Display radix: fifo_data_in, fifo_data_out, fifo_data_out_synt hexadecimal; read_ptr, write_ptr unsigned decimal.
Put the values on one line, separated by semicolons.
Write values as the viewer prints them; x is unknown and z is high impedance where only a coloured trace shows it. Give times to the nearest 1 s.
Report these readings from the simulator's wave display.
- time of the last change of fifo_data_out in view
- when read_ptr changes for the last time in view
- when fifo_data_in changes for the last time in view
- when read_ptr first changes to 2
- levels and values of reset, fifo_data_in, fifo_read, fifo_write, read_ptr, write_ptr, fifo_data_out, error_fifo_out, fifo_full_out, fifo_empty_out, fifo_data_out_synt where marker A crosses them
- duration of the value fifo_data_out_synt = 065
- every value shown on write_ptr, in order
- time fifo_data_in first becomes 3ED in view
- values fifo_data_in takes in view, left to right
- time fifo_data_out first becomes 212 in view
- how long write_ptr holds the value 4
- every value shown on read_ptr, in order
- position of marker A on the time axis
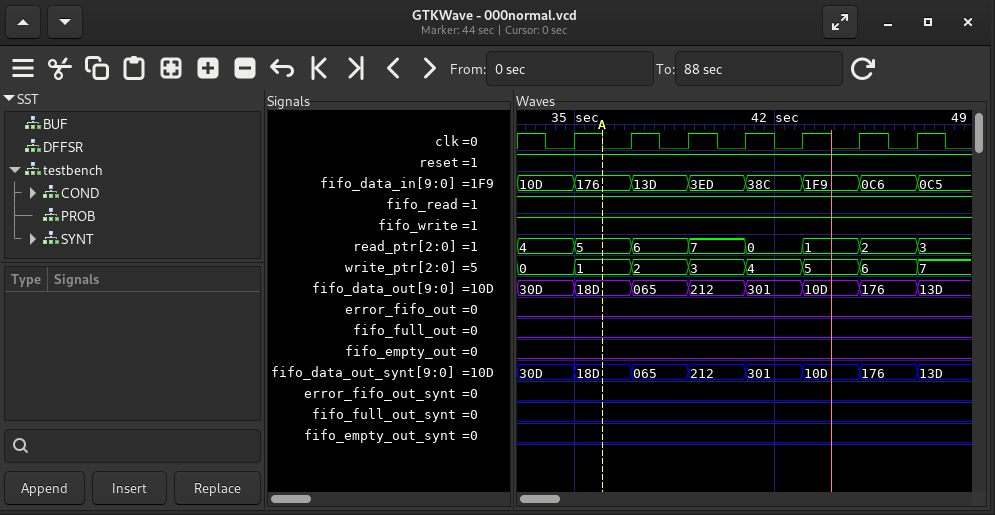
47 s; 47 s; 47 s; 45 s; reset=1, fifo_data_in=176, fifo_read=1, fifo_write=1, read_ptr=5, write_ptr=1, fifo_data_out=18D, error_fifo_out=0, fifo_full_out=0, fifo_empty_out=0, fifo_data_out_synt=18D; 2 s; 0, 1, 2, 3, 4, 5, 6, 7; 39 s; 10D, 176, 13D, 3ED, 38C, 1F9, 0C6, 0C5; 39 s; 2 s; 4, 5, 6, 7, 0, 1, 2, 3; 36 s
